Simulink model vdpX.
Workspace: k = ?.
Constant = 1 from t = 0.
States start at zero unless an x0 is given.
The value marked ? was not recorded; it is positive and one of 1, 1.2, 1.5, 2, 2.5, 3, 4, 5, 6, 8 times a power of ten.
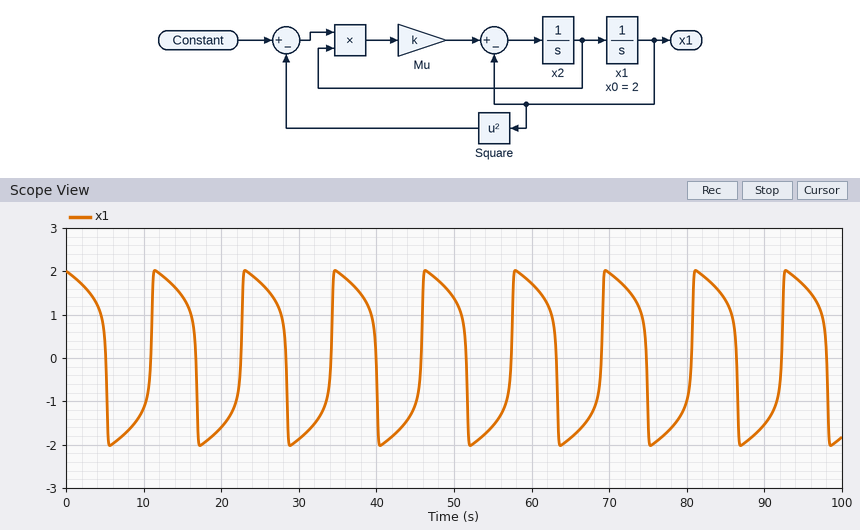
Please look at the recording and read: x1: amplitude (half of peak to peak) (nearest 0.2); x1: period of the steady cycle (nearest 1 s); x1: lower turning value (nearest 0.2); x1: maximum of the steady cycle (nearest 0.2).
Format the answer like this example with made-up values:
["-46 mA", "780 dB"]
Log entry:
["2.0", "12 s", "-2.0", "2.0"]
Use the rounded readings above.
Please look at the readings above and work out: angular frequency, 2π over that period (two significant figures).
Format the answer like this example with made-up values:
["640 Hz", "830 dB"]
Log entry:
["0.52 rad/s"]
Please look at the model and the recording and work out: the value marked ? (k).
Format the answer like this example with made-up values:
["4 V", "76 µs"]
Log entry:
["5"]
